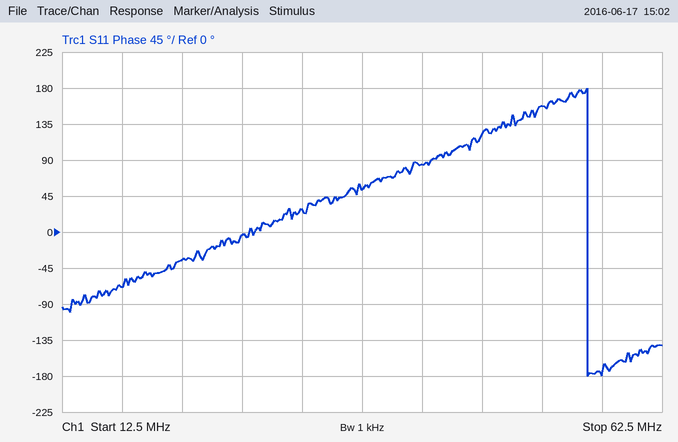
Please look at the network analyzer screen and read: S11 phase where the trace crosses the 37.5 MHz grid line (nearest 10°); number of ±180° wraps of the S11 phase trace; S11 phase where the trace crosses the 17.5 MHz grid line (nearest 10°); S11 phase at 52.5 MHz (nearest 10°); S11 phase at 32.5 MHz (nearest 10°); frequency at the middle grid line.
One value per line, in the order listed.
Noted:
50°
1
-70°
160°
30°
37.5 MHz
